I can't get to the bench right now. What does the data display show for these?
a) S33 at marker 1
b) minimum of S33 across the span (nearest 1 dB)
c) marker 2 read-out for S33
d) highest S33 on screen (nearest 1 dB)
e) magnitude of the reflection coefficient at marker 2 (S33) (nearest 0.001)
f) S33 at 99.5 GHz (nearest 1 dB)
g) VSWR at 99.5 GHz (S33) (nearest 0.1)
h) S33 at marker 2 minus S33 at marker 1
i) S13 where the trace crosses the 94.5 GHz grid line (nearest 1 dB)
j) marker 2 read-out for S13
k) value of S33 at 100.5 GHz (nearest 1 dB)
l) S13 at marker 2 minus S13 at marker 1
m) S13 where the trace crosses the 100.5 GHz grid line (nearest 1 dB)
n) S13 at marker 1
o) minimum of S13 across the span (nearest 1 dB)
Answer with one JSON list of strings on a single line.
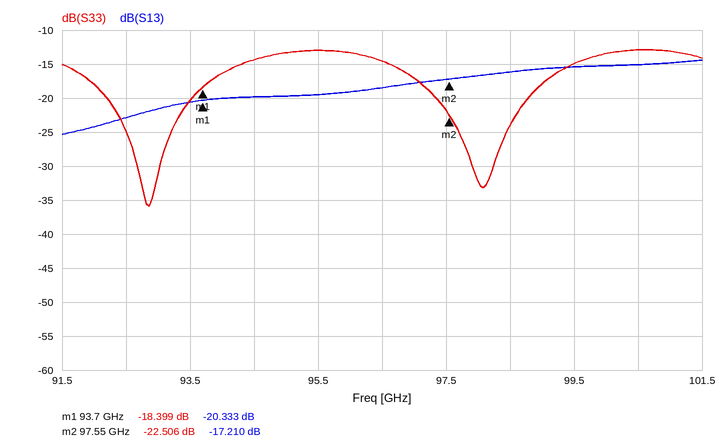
["-18.399 dB", "-36 dB", "-22.506 dB", "-13 dB", "0.075", "-15 dB", "1.4", "-4.107 dB", "-20 dB", "-17.210 dB", "-13 dB", "3.123 dB", "-15 dB", "-20.333 dB", "-25 dB"]
